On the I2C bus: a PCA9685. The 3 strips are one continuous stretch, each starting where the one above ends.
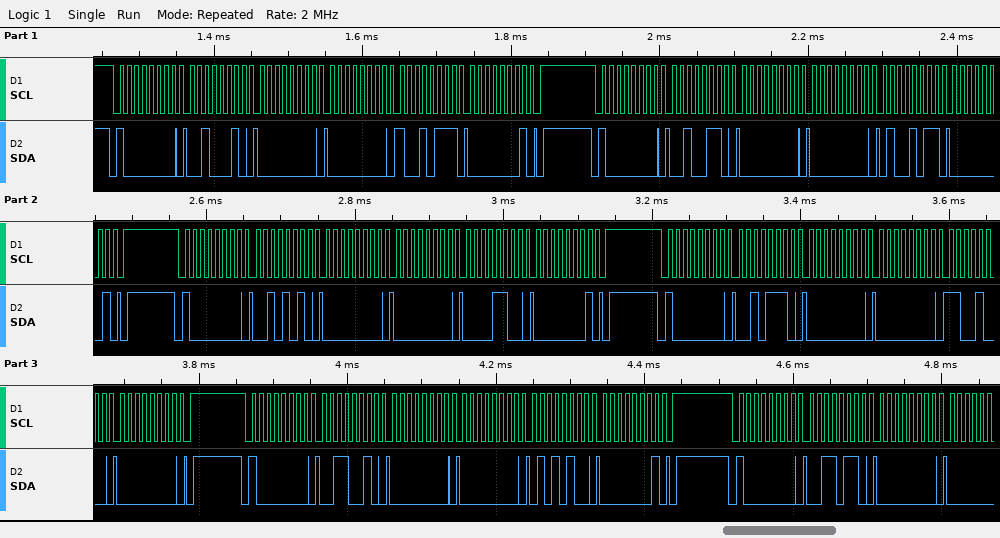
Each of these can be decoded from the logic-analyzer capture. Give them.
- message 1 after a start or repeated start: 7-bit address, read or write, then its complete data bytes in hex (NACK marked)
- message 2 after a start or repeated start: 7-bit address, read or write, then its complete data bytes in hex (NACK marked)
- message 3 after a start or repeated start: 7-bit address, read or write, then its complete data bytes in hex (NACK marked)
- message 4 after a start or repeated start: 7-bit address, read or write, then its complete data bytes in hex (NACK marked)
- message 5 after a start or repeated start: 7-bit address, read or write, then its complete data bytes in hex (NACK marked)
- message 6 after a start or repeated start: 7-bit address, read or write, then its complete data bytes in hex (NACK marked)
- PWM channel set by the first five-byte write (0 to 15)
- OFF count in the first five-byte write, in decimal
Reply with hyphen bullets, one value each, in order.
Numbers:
- 0x40 write: 22 00 00 97 01
- 0x40 write: 26 00 00 4B 01
- 0x40 write: 2A 00 00 0C 01
- 0x40 write: 2E 00 00 C8 00
- 0x40 write: 32 00 00 54 01
- 0x40 write: 36 00
- 7
- 407
